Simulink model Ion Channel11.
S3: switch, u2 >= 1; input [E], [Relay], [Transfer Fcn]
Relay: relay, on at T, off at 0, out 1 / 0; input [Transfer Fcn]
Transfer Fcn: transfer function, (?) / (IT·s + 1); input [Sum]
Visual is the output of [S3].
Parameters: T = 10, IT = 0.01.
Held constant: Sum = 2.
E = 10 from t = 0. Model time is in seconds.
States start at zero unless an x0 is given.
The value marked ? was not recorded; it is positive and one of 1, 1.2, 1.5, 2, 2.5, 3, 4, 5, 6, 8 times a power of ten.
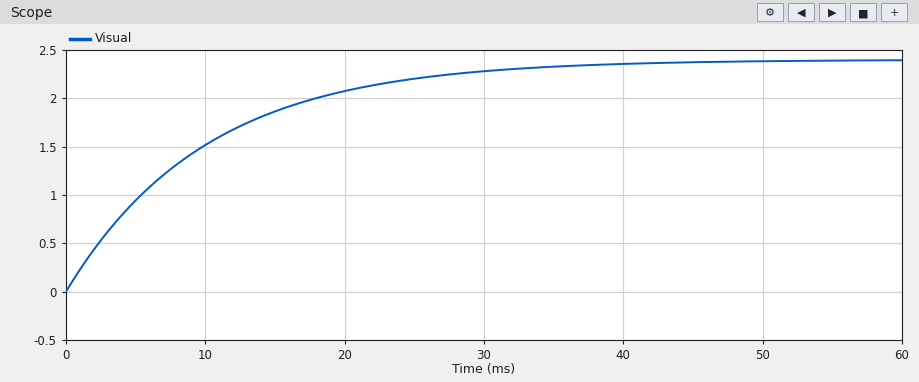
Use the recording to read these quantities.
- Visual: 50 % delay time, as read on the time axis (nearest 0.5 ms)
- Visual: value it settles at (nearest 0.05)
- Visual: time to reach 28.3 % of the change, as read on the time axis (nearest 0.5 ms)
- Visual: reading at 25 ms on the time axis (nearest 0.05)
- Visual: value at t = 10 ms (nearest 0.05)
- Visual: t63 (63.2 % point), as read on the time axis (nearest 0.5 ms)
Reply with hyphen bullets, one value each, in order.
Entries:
- 7.0 ms
- 2.40
- 3.5 ms
- 2.20
- 1.50
- 10.0 ms
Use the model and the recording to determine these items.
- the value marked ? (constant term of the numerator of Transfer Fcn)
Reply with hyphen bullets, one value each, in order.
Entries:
- 1.2
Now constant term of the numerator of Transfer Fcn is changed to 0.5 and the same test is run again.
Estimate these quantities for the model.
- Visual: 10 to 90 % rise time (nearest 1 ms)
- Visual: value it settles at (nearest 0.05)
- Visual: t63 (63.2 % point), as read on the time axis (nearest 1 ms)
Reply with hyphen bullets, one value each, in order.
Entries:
- 22 ms
- 1.00
- 10 ms
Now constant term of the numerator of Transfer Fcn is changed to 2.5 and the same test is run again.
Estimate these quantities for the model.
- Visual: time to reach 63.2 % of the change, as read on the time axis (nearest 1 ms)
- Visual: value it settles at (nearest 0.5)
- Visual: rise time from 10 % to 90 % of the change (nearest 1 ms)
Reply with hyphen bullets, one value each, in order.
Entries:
- 10 ms
- 5.0
- 22 ms
